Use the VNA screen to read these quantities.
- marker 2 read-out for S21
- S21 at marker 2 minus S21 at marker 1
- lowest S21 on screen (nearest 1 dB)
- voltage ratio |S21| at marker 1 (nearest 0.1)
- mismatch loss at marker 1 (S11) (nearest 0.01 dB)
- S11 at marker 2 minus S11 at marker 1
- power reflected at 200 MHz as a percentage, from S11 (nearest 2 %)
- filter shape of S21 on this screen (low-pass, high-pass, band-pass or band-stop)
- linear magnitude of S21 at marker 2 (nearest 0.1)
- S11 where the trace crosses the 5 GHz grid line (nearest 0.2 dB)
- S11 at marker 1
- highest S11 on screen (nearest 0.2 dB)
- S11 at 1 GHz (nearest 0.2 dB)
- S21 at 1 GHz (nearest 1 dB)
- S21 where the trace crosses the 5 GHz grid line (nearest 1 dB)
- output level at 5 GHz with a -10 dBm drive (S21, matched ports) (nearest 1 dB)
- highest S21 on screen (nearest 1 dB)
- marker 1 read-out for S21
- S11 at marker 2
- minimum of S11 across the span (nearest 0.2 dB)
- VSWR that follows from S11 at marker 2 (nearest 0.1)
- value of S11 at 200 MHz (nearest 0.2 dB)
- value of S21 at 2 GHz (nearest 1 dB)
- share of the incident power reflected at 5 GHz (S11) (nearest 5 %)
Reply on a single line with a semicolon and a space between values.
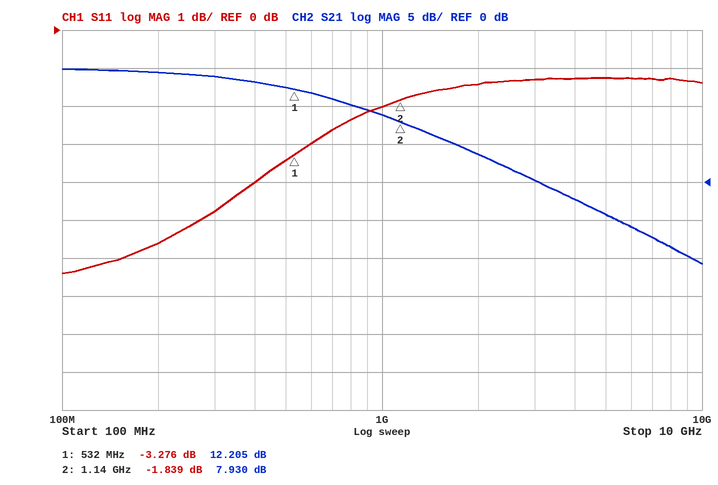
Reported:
7.930 dB; -4.275 dB; -11 dB; 4.1; 2.76 dB; 1.437 dB; 28 %; low-pass; 2.5; -1.2 dB; -3.276 dB; -1.2 dB; -2.0 dB; 9 dB; -4 dB; -14 dBm; 15 dB; 12.205 dB; -1.839 dB; -6.4 dB; 9.5; -5.6 dB; 4 dB; 75 %
